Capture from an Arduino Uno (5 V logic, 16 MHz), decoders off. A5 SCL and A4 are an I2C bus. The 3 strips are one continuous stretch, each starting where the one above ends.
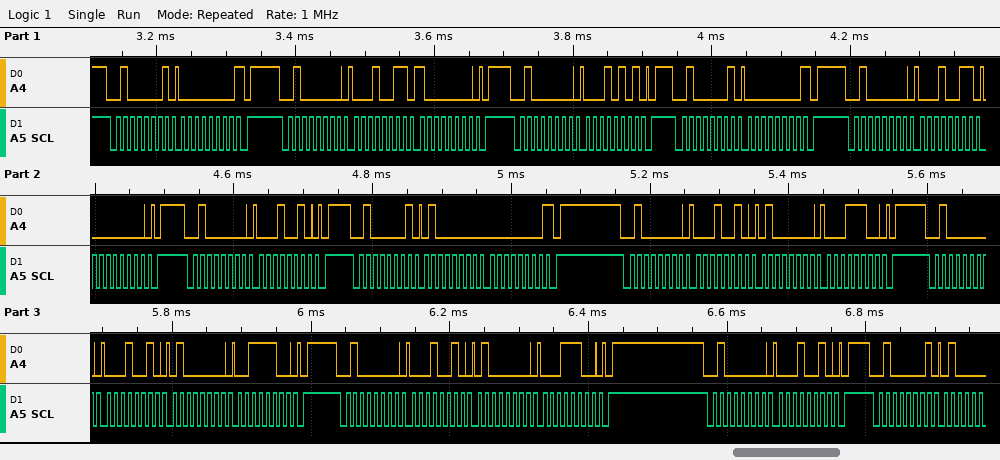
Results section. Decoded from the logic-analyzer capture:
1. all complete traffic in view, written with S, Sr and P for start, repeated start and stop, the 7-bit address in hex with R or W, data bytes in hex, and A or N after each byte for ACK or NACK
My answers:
S 20R A 00 N P S 20W A 13 A 80 A P S 20W A 15 A P S 20R A 00 N P S 20W A 13 A 00 A P S 20W A 12 A P S 20R A 40 A 00 N P S 20W A 12 A 40 A 1C A P S 20W A 12 A 40 A 3C A P S 20W A 12 A 40 A 1C A P S 20W A 12 A P S 20R A
